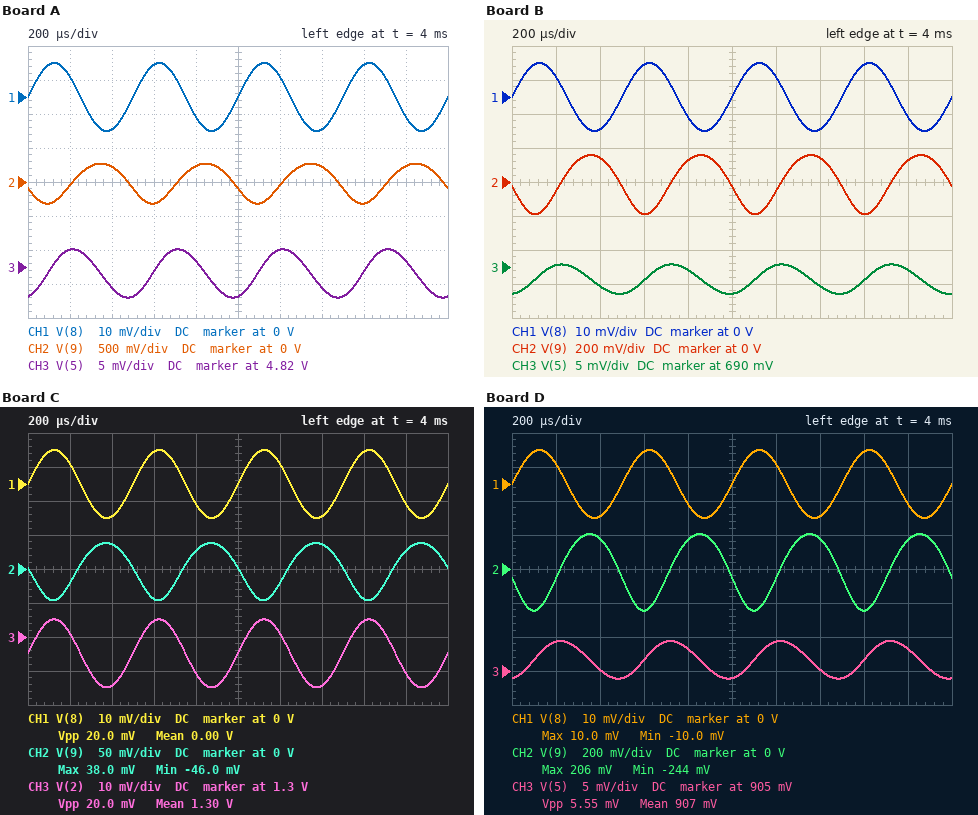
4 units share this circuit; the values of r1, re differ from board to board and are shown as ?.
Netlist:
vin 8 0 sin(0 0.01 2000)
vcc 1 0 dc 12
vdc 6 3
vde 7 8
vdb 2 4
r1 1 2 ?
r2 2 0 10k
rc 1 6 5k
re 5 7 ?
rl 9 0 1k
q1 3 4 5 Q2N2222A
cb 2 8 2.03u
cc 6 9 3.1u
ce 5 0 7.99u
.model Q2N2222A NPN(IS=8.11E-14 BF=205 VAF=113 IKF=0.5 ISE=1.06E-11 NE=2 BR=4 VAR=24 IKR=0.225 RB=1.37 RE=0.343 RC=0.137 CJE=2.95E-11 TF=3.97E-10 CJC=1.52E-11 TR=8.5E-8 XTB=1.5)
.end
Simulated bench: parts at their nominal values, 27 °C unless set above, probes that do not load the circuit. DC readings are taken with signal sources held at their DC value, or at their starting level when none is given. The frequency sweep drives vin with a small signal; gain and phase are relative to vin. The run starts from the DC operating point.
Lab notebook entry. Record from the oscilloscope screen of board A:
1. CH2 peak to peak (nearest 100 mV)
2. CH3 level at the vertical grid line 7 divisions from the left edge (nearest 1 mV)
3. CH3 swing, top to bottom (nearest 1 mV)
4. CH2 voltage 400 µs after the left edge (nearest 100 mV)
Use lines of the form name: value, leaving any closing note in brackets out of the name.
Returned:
CH2 peak to peak: 600 mV
CH3 level at the vertical grid line 7 divisions from the left edge: 4.817 V
CH3 swing, top to bottom: 7 mV
CH2 voltage 400 µs after the left edge: 200 mV
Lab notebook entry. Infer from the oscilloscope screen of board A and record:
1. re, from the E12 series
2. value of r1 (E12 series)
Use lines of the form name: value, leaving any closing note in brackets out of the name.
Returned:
re, from the E12 series: 4.7 kΩ
value of r1: 12 kΩ
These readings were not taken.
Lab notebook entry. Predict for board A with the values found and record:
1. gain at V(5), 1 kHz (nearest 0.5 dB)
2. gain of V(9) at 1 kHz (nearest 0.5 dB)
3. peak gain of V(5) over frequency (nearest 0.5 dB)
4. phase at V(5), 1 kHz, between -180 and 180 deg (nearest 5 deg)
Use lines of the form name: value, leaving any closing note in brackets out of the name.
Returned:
gain at V(5), 1 kHz: -4.5 dB
gain of V(9) at 1 kHz: 28.0 dB
peak gain of V(5) over frequency: -0.5 dB
phase at V(5), 1 kHz, between -180 and 180 deg: -50 deg
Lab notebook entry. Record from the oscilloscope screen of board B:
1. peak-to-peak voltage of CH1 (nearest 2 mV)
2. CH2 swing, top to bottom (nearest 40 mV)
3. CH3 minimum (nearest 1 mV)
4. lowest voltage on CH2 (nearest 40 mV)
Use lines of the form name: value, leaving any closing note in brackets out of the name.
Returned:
peak-to-peak voltage of CH1: 20 mV
CH2 swing, top to bottom: 360 mV
CH3 minimum: 686 mV
lowest voltage on CH2: -200 mV
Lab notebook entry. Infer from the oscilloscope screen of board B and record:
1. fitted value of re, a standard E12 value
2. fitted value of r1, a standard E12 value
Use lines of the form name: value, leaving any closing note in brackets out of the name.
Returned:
fitted value of re, a standard E12 value: 1.2 kΩ
fitted value of r1, a standard E12 value: 82 kΩ
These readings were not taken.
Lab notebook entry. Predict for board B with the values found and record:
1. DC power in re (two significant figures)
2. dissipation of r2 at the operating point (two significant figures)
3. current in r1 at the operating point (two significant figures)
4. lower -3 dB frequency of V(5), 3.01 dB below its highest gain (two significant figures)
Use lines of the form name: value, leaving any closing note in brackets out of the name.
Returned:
DC power in re: 390 µW
dissipation of r2 at the operating point: 160 µW
current in r1 at the operating point: 130 µA
lower -3 dB frequency of V(5), 3.01 dB below its highest gain: 8.6 Hz
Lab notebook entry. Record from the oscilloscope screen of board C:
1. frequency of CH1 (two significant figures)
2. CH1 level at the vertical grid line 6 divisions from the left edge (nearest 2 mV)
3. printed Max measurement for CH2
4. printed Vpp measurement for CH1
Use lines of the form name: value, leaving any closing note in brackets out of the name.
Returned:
frequency of CH1: 2.0 kHz
CH1 level at the vertical grid line 6 divisions from the left edge: 6 mV
printed Max measurement for CH2: 38.0 mV
printed Vpp measurement for CH1: 20.0 mV
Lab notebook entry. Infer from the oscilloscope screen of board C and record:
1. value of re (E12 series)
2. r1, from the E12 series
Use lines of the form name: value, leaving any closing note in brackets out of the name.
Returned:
value of re: 5.6 kΩ
r1, from the E12 series: 82 kΩ
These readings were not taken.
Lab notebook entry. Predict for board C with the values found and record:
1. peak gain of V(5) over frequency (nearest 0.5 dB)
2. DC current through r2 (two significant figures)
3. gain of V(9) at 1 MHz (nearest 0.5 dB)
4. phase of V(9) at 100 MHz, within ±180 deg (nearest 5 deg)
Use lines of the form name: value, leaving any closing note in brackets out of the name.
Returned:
peak gain of V(5) over frequency: -1.0 dB
DC current through r2: 130 µA
gain of V(9) at 1 MHz: 12.5 dB
phase of V(9) at 100 MHz, within ±180 deg: 65 deg
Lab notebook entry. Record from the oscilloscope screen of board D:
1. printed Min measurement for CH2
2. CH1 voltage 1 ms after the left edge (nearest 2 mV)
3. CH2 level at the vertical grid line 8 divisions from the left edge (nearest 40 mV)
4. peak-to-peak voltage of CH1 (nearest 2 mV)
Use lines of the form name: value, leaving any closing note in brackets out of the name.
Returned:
printed Min measurement for CH2: -244 mV
CH1 voltage 1 ms after the left edge: 0 V
CH2 level at the vertical grid line 8 divisions from the left edge: -240 mV
peak-to-peak voltage of CH1: 20 mV
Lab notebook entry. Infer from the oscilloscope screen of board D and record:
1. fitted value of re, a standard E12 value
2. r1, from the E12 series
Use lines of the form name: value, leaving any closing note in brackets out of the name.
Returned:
fitted value of re, a standard E12 value: 1.2 kΩ
r1, from the E12 series: 68 kΩ
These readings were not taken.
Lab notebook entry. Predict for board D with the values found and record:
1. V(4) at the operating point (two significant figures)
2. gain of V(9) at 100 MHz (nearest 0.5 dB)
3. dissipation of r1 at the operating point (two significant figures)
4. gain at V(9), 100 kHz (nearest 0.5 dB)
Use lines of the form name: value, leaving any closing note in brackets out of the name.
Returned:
V(4) at the operating point: 1.5 V
gain of V(9) at 100 MHz: 15.5 dB
dissipation of r1 at the operating point: 1.6 mW
gain at V(9), 100 kHz: 27.5 dB
